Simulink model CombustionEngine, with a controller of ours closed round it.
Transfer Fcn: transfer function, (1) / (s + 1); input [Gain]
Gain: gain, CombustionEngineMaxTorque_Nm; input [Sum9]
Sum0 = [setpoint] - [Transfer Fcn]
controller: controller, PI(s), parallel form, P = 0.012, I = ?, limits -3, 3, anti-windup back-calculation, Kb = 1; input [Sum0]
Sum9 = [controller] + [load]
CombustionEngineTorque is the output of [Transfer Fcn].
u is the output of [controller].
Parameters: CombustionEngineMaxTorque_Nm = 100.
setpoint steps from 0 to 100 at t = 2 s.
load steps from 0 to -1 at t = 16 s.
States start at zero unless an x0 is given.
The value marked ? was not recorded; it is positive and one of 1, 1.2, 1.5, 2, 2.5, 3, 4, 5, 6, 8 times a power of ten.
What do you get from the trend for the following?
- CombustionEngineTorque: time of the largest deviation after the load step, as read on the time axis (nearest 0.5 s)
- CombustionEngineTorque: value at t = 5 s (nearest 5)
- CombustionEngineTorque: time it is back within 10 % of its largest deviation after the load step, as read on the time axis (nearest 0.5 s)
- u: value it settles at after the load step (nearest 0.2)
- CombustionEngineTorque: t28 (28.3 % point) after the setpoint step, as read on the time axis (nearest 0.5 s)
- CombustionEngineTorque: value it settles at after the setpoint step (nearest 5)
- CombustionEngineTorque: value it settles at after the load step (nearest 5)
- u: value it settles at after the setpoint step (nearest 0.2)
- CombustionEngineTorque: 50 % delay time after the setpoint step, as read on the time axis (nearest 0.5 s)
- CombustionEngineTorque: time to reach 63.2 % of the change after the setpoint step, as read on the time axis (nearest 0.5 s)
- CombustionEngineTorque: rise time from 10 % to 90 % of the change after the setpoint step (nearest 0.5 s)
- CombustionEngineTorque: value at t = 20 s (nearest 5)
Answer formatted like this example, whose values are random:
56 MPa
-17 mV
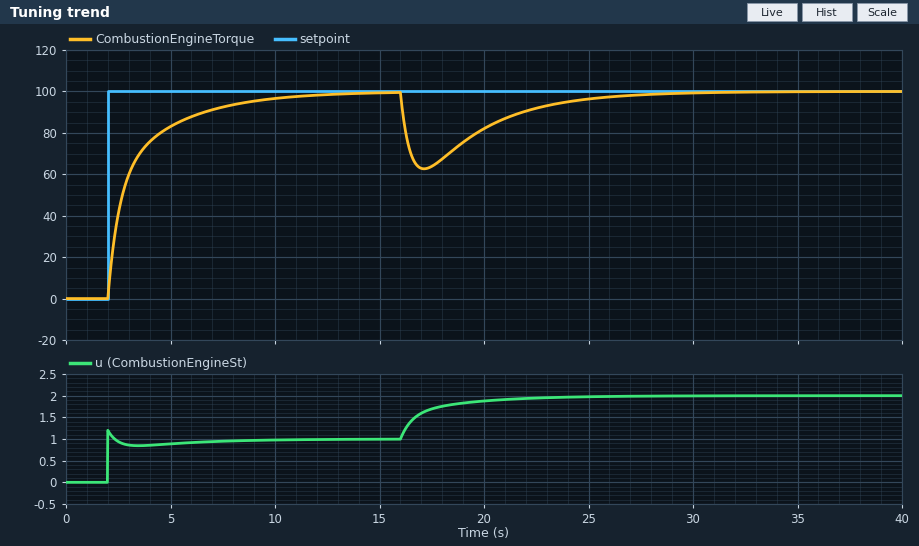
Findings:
17.0 s
85
25.0 s
2.0
2.5 s
100
100
1.0
2.5 s
3.0 s
4.5 s
80
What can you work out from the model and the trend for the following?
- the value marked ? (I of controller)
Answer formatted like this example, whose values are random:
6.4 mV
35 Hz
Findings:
0.006
